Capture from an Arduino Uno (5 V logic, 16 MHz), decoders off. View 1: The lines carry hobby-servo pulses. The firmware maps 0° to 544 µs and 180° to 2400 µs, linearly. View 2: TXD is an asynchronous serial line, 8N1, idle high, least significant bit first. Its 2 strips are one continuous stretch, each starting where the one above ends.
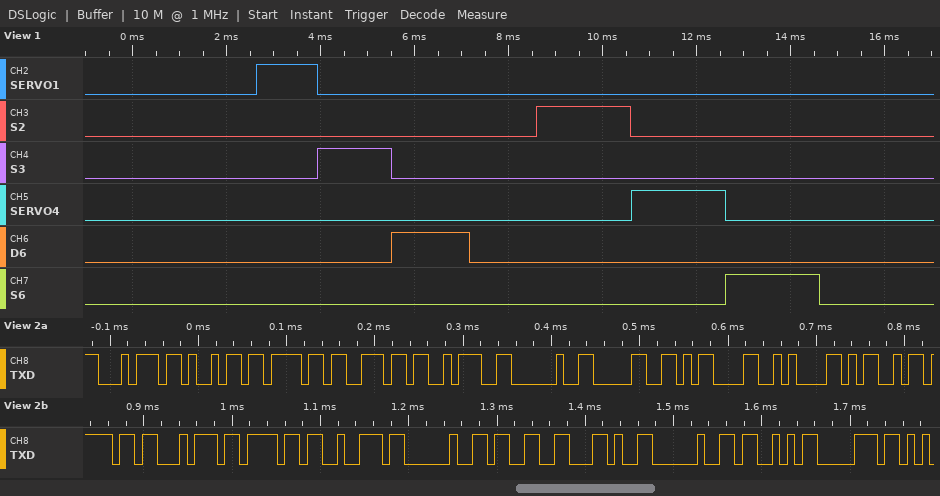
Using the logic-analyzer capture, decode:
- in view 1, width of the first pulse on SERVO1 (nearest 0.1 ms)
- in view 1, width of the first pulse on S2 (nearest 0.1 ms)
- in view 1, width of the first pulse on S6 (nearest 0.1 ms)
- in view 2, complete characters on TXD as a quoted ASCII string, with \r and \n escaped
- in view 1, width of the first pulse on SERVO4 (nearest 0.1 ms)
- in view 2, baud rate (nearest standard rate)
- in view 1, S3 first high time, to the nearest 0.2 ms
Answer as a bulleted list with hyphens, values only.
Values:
- 1.3 ms
- 2.0 ms
- 2.0 ms
- "tion: 0\r\nMotor 3, Sp"
- 2.0 ms
- 115200 baud
- 1.6 ms
